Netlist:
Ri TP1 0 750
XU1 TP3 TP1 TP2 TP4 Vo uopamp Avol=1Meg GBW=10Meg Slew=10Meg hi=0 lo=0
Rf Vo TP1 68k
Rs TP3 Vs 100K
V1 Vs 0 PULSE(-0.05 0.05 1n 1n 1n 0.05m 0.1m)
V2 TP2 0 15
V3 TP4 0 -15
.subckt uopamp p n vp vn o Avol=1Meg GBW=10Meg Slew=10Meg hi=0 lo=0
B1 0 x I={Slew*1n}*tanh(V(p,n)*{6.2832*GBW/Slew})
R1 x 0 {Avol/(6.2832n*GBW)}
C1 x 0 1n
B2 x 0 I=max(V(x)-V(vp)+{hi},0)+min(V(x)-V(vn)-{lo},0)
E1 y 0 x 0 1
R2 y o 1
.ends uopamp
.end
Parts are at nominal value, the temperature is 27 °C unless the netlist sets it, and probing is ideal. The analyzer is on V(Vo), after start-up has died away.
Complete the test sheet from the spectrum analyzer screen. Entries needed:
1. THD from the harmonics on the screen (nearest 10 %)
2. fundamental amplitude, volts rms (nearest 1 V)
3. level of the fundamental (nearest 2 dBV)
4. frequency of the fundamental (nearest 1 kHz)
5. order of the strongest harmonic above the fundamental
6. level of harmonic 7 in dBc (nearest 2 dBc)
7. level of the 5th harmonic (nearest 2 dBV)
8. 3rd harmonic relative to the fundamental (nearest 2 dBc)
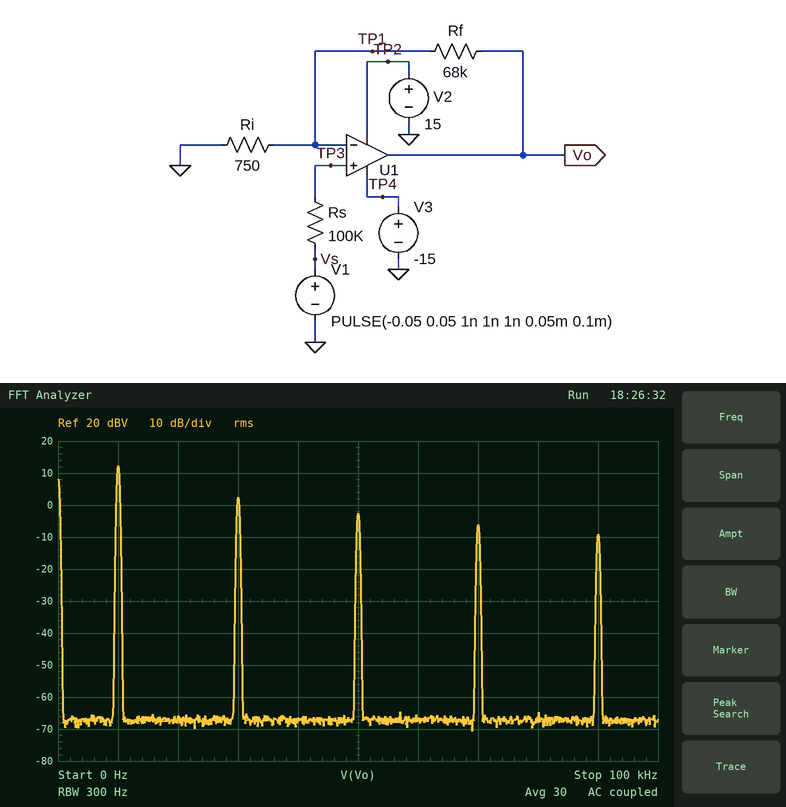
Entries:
40 %
4 V
12 dBV
10 kHz
3
-18 dBc
-2 dBV
-10 dBc
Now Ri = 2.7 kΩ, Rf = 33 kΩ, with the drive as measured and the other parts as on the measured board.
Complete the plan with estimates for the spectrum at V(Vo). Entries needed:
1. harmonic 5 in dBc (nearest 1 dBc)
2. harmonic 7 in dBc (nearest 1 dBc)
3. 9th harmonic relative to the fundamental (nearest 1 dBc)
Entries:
-14 dBc
-17 dBc
-19 dBc
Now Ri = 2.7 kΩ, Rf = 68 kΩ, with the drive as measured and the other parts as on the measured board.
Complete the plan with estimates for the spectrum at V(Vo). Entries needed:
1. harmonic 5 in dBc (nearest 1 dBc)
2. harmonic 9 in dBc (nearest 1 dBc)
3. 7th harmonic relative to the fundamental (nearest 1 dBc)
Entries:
-14 dBc
-19 dBc
-17 dBc
